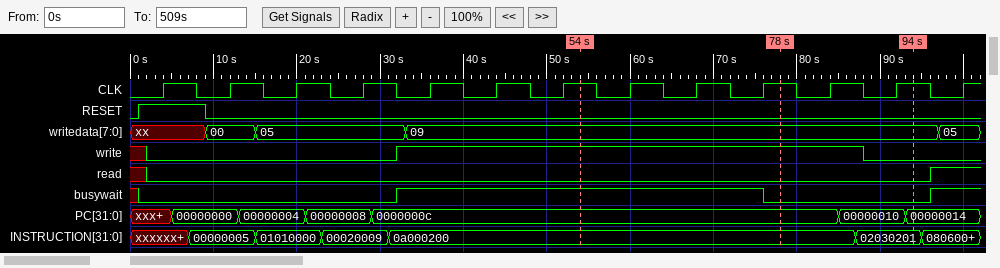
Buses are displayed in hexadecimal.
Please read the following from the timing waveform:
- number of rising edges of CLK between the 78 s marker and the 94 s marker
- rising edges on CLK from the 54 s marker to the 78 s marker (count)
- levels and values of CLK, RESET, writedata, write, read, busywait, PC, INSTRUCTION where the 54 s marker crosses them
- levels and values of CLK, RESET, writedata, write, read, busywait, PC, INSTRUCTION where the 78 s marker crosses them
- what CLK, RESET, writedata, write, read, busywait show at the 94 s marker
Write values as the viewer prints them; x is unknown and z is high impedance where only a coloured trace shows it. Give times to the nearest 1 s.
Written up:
2
3
CLK=1, RESET=0, writedata=09, write=1, read=0, busywait=1, PC=0000000c, INSTRUCTION=0a000200
CLK=1, RESET=0, writedata=09, write=1, read=0, busywait=0, PC=0000000c, INSTRUCTION=0a000200
CLK=1, RESET=0, writedata=09, write=0, read=0, busywait=0
